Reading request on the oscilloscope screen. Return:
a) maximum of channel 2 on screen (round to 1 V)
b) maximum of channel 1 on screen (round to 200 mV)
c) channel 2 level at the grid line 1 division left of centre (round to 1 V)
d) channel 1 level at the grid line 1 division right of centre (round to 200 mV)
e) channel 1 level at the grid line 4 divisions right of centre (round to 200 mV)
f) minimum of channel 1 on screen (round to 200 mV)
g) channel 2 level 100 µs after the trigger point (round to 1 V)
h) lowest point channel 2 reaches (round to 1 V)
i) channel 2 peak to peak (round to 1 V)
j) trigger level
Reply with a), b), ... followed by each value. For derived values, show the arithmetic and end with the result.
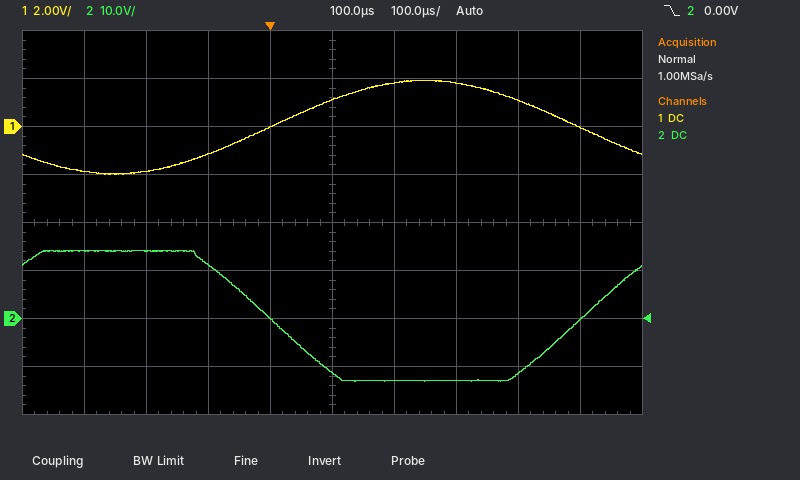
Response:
a) 14 V
b) 2.0 V
c) 0 V
d) 1.8 V
e) 0.0 V
f) -2.0 V
g) -11 V
h) -13 V
i) 14 V − (-13 V) = 27 V
j) 0.00 V
